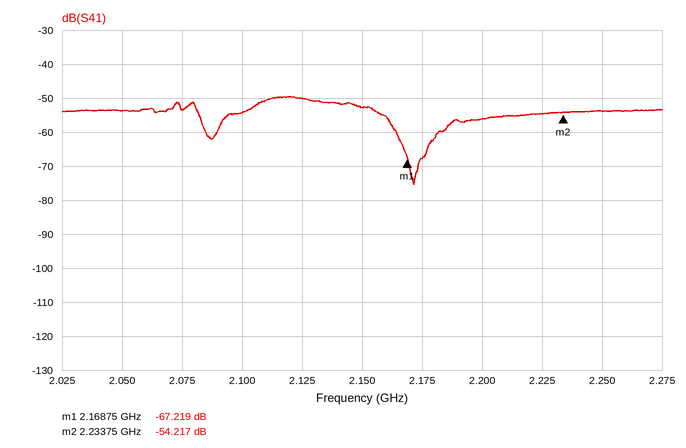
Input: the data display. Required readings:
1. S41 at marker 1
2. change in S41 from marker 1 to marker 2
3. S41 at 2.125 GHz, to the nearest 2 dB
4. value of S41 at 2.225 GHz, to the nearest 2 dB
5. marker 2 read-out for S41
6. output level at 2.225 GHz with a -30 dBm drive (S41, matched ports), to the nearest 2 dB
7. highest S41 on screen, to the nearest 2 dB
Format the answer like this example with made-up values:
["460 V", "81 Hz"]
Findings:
["-67.219 dB", "13.002 dB", "-50 dB", "-54 dB", "-54.217 dB", "-84 dBm", "-50 dB"]
